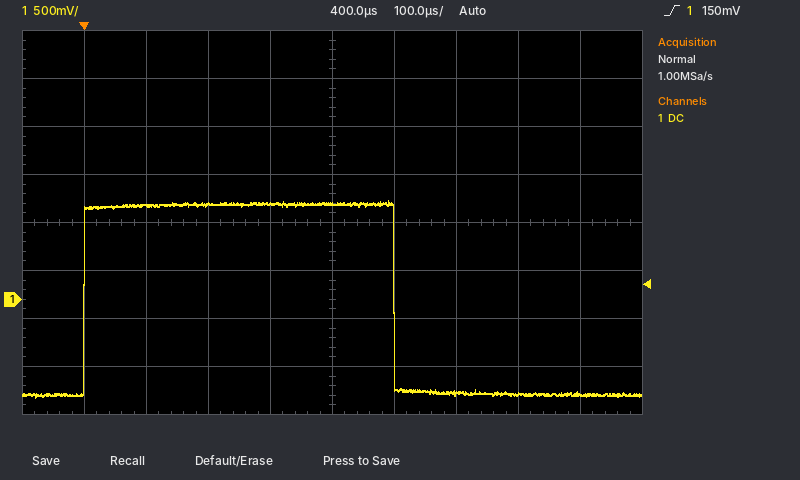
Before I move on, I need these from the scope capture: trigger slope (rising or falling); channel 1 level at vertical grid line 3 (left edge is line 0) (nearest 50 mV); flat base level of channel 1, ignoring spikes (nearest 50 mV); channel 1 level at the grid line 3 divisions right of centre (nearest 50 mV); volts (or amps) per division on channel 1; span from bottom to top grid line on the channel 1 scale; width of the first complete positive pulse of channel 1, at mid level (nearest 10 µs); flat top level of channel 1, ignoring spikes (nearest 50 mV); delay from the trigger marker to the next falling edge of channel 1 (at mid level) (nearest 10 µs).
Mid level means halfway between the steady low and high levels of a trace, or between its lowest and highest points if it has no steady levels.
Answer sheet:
rising
1.00 V
-1.00 V
-1.00 V
500 mV
4 V
500 µs
1.00 V
500 µs
